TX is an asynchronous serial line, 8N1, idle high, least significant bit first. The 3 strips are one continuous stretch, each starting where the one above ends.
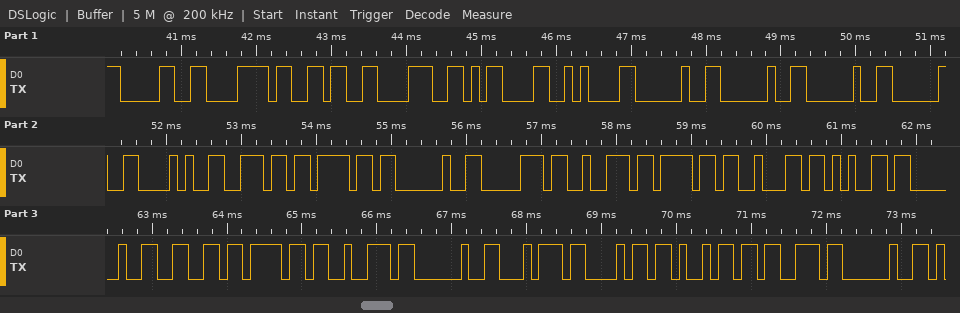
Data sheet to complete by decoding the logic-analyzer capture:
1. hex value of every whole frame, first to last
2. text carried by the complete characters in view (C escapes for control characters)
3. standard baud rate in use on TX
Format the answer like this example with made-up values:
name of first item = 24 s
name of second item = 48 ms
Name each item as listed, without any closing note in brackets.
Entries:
hex value of every whole frame, first to last = 30 78 36 38 0D 0A 20 20 20 20 28 6E 6F 20 70 72 6F 62 65 20 66 6F 72 20 74 68 69 73 20
text carried by the complete characters in view = "0x68\r\n    (no probe for this "
standard baud rate in use on TX = 9600 baud
